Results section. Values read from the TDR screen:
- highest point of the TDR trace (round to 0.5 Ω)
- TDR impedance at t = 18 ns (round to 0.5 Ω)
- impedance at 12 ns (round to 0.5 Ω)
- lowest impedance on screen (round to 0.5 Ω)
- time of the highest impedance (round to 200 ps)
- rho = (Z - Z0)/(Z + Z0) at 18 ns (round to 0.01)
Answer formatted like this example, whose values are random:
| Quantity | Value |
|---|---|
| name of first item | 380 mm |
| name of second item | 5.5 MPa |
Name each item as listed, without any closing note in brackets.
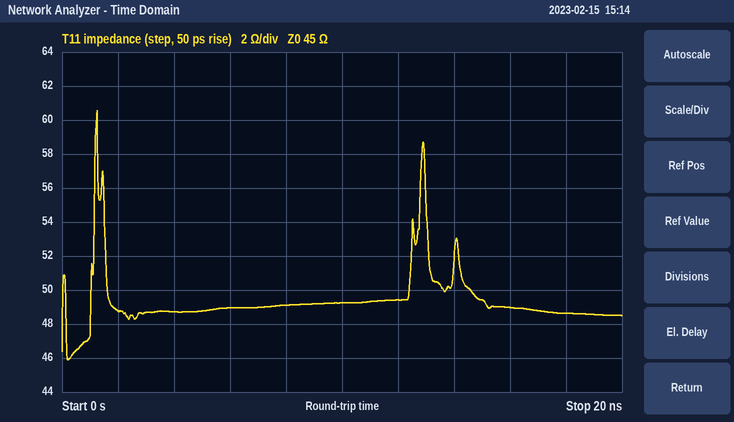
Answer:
| Quantity | Value |
|---|---|
| highest point of the TDR trace | 60.5 Ω |
| TDR impedance at t = 18 ns | 48.5 Ω |
| impedance at 12 ns | 49.5 Ω |
| lowest impedance on screen | 46.0 Ω |
| time of the highest impedance | 1.2 ns |
| rho = (Z - Z0)/(Z + Z0) at 18 ns | +0.04 |
